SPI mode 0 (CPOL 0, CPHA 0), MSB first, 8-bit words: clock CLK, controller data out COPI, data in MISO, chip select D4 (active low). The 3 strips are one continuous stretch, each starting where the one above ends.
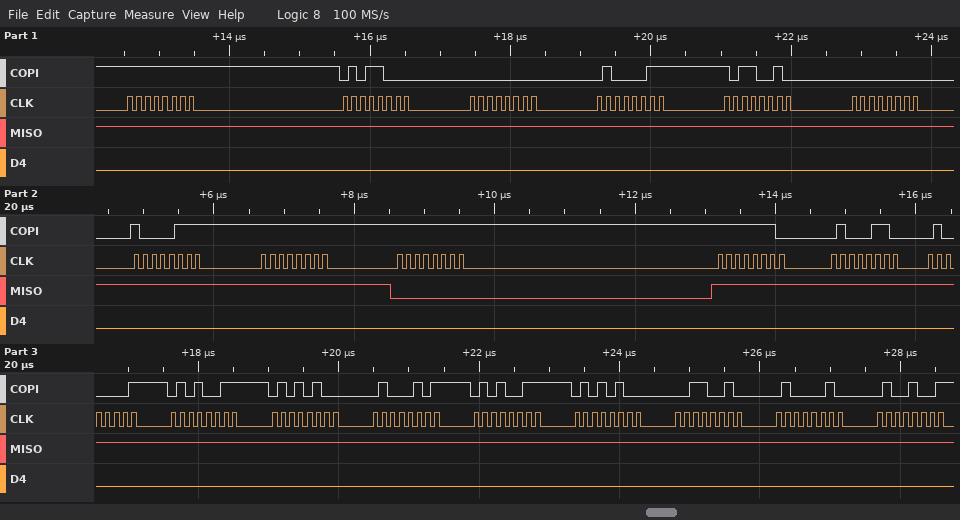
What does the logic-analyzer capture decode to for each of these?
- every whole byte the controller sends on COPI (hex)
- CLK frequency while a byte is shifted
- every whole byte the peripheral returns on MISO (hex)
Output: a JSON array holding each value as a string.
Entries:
["0xFF 0x58 0x00 0x43 0xB2 0x00 0x87 0xFF 0xFF 0xFE 0x46 0x41 0x53 0x54 0x45 0x53 0x54 0x32 0x42 0x49", "8 MHz", "0xFF 0xFF 0xFF 0xFF 0xFF 0xFF 0xFF 0xFF 0x00 0xFF 0xFF 0xFF 0xFF 0xFF 0xFF 0xFF 0xFF 0xFF 0xFF 0xFF"]
